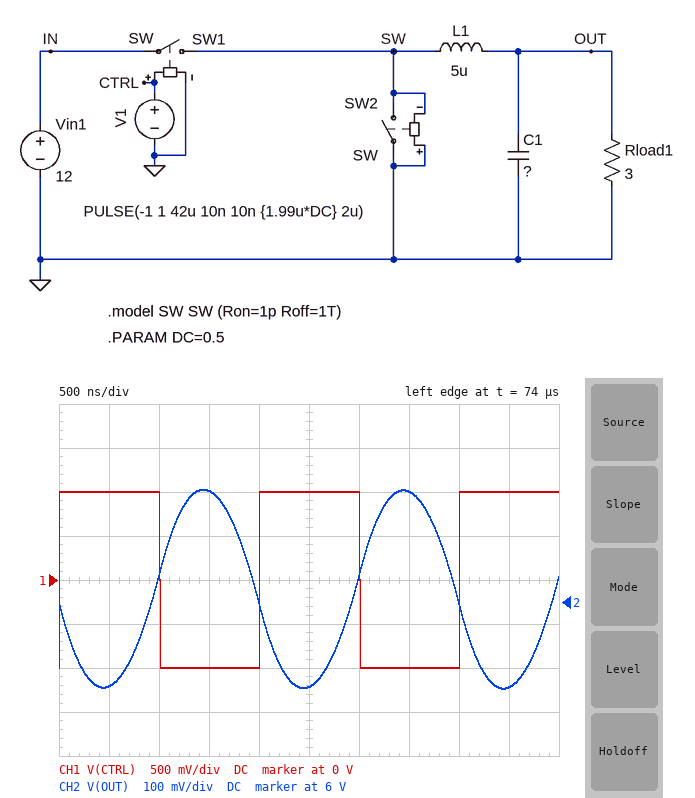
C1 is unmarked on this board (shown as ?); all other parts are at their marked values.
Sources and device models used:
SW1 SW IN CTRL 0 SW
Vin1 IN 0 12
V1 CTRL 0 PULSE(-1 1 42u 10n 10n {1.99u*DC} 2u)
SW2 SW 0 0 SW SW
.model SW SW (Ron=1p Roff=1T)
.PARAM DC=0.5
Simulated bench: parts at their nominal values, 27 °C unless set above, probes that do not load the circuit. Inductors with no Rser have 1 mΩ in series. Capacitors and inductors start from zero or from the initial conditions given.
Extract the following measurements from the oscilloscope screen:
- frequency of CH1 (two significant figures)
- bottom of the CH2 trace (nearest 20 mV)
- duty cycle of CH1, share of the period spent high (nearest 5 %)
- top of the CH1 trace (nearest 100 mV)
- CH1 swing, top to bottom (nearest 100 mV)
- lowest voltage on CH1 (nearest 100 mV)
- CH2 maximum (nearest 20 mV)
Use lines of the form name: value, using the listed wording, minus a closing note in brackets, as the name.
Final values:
frequency of CH1: 500 kHz
bottom of the CH2 trace: 5.80 V
duty cycle of CH1, share of the period spent high: 50 %
top of the CH1 trace: 1.0 V
CH1 swing, top to bottom: 2.0 V
lowest voltage on CH1: -1.0 V
CH2 maximum: 6.26 V
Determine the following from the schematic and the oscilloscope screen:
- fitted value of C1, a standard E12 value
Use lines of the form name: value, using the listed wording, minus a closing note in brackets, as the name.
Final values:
fitted value of C1, a standard E12 value: 680 nF
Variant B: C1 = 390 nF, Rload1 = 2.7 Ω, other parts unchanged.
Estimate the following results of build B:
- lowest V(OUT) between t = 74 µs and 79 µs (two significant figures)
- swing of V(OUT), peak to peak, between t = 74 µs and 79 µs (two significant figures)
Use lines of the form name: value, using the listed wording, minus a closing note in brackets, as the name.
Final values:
lowest V(OUT) between t = 74 µs and 79 µs: 5.6 V
swing of V(OUT), peak to peak, between t = 74 µs and 79 µs: 780 mV
